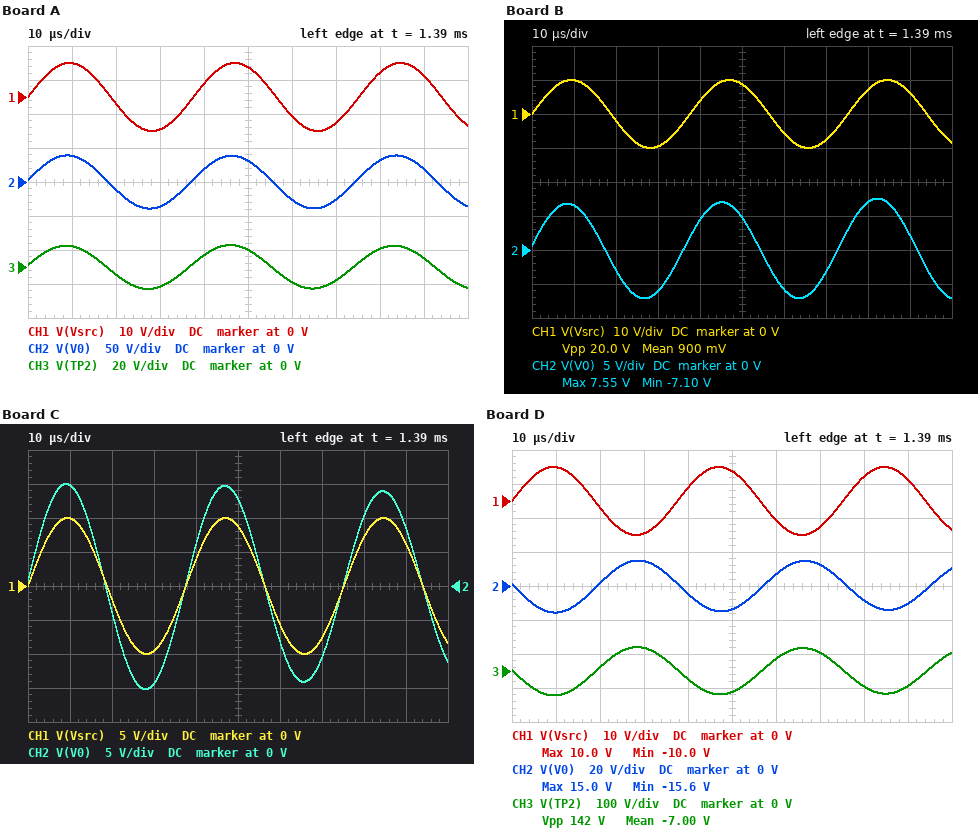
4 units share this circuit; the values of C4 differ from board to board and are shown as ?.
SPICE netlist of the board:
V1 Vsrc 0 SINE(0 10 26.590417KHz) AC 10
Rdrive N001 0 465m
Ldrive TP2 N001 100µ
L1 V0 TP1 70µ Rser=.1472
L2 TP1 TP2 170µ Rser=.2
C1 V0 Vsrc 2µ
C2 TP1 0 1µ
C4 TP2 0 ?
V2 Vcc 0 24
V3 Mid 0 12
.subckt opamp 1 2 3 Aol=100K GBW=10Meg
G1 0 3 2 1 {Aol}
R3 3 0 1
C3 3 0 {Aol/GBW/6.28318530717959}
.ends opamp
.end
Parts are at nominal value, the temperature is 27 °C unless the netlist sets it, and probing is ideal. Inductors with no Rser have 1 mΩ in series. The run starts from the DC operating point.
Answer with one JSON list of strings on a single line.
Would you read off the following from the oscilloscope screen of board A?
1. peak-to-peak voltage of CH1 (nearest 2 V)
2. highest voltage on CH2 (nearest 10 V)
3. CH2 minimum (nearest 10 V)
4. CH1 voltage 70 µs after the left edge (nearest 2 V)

["20 V", "40 V", "-40 V", "-8 V"]
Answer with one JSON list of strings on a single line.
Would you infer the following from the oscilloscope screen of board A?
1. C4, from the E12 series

["1.8 µF"]
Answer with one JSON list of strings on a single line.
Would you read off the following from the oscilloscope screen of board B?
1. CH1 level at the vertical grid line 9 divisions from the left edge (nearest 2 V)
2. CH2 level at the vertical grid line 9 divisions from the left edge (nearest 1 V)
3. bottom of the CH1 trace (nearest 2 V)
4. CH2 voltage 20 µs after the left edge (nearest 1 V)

["6 V", "2 V", "-10 V", "-3 V"]
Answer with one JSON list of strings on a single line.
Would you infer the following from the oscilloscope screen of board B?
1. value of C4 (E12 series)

["680 nF"]
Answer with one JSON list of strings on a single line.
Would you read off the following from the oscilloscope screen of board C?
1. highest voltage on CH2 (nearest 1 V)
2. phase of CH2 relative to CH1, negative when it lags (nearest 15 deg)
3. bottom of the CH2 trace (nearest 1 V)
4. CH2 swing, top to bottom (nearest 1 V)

["15 V", "0 deg", "-15 V", "30 V"]
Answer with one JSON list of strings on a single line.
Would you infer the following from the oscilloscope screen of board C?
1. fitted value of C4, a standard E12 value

["560 nF"]
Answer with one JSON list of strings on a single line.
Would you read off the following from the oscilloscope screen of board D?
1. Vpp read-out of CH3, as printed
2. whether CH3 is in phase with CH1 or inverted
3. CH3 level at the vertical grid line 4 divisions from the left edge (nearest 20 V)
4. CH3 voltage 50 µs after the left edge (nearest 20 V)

["142 V", "inverted", "-20 V", "-60 V"]
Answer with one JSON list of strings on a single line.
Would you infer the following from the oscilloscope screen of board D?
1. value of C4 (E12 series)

["820 nF"]
